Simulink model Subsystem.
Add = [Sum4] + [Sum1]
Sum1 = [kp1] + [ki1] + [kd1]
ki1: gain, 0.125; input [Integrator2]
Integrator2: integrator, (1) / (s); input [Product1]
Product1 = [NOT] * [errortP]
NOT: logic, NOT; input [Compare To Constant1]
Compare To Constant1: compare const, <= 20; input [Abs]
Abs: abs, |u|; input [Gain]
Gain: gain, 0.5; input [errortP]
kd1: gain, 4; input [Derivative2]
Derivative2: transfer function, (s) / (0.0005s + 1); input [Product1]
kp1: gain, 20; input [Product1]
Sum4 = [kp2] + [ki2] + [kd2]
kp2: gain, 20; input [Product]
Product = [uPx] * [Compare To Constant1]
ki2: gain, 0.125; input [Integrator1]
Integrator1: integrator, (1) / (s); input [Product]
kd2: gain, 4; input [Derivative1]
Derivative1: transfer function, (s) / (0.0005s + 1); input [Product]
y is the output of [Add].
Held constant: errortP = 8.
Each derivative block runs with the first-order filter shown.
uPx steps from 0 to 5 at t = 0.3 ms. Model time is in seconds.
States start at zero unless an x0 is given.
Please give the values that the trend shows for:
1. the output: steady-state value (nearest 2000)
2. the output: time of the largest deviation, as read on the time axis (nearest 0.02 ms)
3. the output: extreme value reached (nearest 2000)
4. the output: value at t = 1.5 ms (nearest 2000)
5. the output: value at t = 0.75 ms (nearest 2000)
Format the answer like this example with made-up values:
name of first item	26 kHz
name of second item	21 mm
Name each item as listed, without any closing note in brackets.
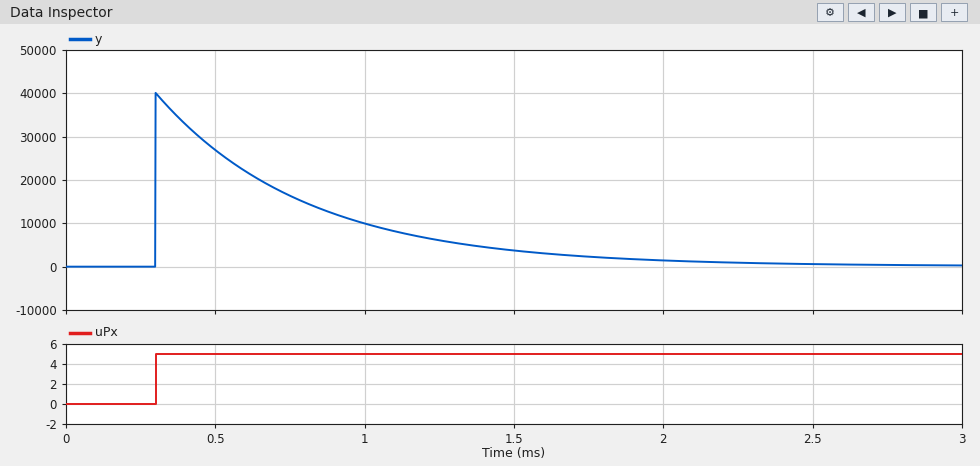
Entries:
the output: steady-state value	0
the output: time of the largest deviation, as read on the time axis	0.30 ms
the output: extreme value reached	40000
the output: value at t = 1.5 ms	4000
the output: value at t = 0.75 ms	16000
